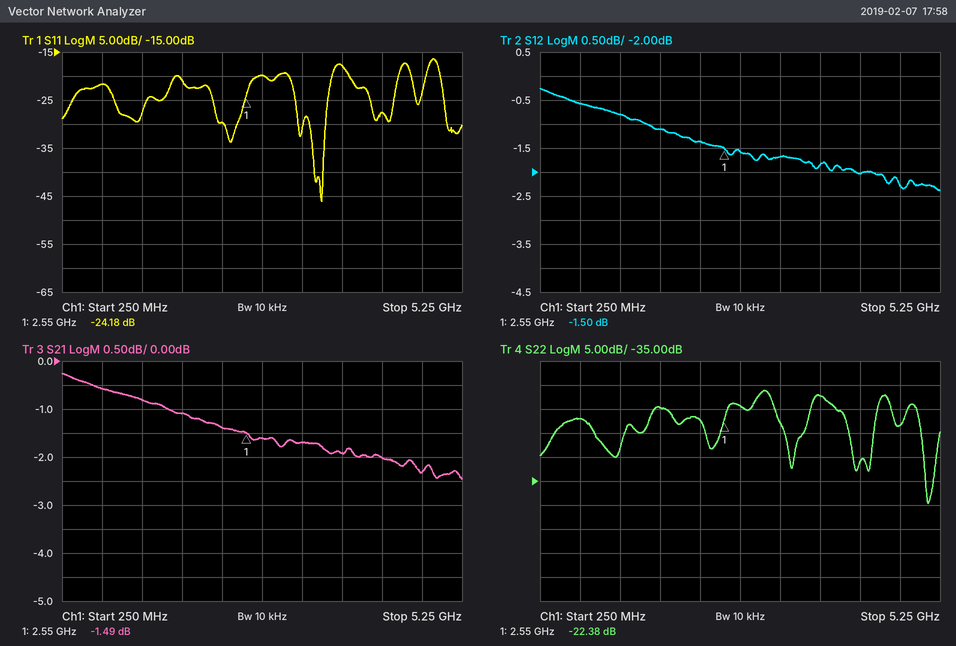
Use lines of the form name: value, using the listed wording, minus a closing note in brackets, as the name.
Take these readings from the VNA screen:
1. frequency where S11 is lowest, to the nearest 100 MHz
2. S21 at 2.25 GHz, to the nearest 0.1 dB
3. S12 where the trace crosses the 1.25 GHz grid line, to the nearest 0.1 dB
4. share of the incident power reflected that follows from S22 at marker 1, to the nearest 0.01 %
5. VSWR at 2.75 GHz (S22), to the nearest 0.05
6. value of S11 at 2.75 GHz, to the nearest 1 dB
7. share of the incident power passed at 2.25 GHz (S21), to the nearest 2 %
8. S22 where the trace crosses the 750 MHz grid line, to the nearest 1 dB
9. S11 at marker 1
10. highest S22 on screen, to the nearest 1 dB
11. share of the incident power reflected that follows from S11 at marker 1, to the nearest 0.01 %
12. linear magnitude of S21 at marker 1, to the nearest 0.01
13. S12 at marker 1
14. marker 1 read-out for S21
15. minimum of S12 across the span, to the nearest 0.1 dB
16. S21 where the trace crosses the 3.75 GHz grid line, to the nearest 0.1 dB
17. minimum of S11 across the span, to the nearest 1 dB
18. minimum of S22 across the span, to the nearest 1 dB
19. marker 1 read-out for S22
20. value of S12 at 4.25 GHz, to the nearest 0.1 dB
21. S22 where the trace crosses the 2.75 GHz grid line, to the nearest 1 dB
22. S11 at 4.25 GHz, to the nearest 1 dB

frequency where S11 is lowest, to the nearest 100 MHz: 3.5 GHz
S21 at 2.25 GHz, to the nearest 0.1 dB: -1.4 dB
S12 where the trace crosses the 1.25 GHz grid line, to the nearest 0.1 dB: -0.8 dB
share of the incident power reflected that follows from S22 at marker 1, to the nearest 0.01 %: 0.58 %
VSWR at 2.75 GHz (S22), to the nearest 0.05: 1.25
value of S11 at 2.75 GHz, to the nearest 1 dB: -20 dB
share of the incident power passed at 2.25 GHz (S21), to the nearest 2 %: 72 %
S22 where the trace crosses the 750 MHz grid line, to the nearest 1 dB: -22 dB
S11 at marker 1: -24.18 dB
highest S22 on screen, to the nearest 1 dB: -16 dB
share of the incident power reflected that follows from S11 at marker 1, to the nearest 0.01 %: 0.38 %
linear magnitude of S21 at marker 1, to the nearest 0.01: 0.84
S12 at marker 1: -1.50 dB
marker 1 read-out for S21: -1.49 dB
minimum of S12 across the span, to the nearest 0.1 dB: -2.4 dB
S21 where the trace crosses the 3.75 GHz grid line, to the nearest 0.1 dB: -1.9 dB
minimum of S11 across the span, to the nearest 1 dB: -46 dB
minimum of S22 across the span, to the nearest 1 dB: -40 dB
marker 1 read-out for S22: -22.38 dB
value of S12 at 4.25 GHz, to the nearest 0.1 dB: -2.0 dB
S22 where the trace crosses the 2.75 GHz grid line, to the nearest 1 dB: -19 dB
S11 at 4.25 GHz, to the nearest 1 dB: -28 dB
